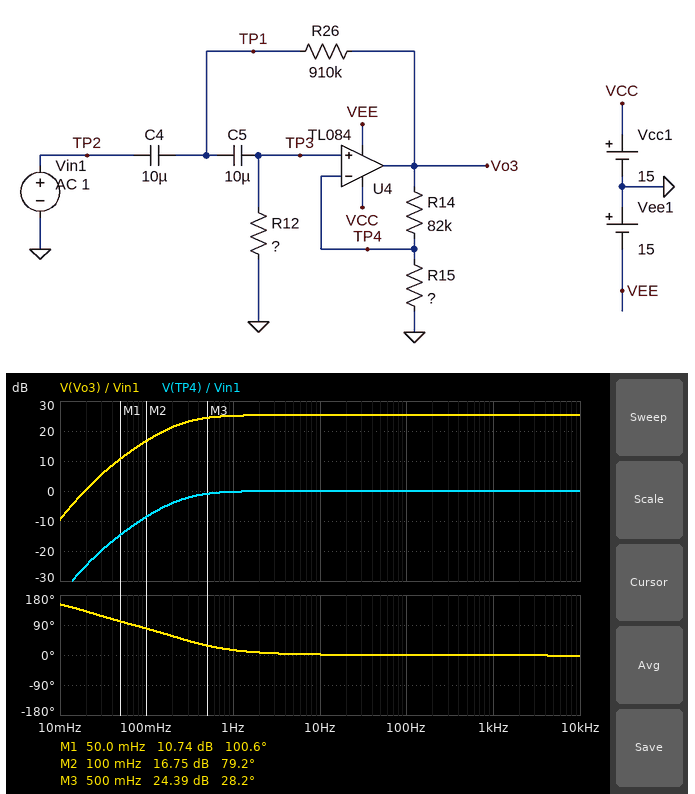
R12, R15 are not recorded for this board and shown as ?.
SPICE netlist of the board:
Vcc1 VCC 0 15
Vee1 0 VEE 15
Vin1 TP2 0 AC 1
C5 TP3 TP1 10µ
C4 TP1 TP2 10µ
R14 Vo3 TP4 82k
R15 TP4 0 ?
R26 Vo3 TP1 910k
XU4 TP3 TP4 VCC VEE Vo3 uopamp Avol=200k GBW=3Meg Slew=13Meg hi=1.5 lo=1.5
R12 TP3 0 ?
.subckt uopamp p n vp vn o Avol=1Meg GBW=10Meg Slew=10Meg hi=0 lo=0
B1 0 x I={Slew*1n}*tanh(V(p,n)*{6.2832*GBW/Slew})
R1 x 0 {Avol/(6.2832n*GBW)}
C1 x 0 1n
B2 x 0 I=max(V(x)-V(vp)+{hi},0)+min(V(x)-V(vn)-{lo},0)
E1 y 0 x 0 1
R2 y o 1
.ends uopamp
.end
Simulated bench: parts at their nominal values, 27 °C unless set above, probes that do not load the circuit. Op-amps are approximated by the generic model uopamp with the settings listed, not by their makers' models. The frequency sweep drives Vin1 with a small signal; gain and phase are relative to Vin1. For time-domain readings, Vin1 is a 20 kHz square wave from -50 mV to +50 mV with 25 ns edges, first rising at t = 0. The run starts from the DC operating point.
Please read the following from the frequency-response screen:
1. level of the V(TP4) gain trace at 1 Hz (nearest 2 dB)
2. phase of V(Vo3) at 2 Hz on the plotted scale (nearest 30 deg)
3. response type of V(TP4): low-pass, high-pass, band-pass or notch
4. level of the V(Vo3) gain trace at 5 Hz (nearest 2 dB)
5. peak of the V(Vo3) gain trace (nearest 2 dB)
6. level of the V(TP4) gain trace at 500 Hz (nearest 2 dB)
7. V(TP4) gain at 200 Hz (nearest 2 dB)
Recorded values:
0 dB
0 deg
high-pass
26 dB
26 dB
0 dB
0 dB
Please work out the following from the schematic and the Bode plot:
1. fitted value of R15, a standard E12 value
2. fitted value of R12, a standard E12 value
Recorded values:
4.7 kΩ
56 kΩ
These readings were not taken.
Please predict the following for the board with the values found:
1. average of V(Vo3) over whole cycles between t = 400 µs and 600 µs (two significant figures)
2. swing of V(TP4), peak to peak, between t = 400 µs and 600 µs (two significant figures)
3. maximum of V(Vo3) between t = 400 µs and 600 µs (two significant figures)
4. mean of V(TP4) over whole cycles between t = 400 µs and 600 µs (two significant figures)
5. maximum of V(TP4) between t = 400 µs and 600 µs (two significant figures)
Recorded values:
920 mV
100 mV
1.8 V
50 mV
100 mV
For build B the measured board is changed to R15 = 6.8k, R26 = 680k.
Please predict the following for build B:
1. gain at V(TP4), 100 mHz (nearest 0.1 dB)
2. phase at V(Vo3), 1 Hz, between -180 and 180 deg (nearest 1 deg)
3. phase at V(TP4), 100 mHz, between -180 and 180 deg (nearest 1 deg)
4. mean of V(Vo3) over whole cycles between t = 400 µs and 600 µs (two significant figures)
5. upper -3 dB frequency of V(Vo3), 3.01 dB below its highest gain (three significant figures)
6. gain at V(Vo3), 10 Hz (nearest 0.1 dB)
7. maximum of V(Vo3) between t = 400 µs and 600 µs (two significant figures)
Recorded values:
-9.2 dB
16 deg
83 deg
650 mV
230 kHz
22.3 dB
1.3 V
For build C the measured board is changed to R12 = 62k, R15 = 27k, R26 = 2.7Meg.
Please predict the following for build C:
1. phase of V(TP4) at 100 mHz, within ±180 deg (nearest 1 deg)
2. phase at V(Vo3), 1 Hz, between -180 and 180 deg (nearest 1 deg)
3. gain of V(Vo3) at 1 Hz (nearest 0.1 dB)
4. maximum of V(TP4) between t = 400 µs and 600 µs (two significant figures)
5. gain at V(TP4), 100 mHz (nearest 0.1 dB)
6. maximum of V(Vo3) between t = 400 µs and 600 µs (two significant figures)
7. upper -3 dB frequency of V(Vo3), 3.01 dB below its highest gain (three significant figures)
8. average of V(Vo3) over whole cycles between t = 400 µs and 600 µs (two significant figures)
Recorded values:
80 deg
26 deg
11.2 dB
100 mV
-14.0 dB
400 mV
743 kHz
200 mV
